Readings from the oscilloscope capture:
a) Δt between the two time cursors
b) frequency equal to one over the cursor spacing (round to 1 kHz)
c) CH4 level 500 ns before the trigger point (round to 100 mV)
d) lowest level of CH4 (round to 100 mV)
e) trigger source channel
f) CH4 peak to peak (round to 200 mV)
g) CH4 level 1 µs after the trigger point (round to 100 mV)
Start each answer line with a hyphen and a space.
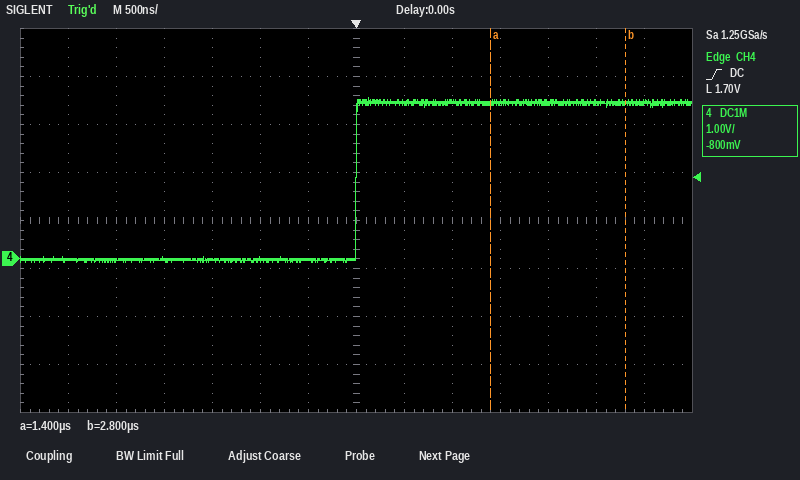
- 1.40 µs
- 714 kHz
- 0.0 V
- -100 mV
- CH4
- 3.4 V
- 3.3 V
